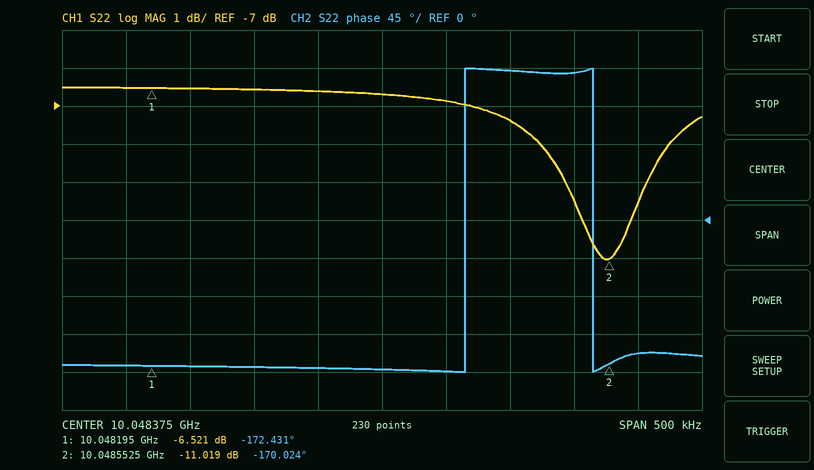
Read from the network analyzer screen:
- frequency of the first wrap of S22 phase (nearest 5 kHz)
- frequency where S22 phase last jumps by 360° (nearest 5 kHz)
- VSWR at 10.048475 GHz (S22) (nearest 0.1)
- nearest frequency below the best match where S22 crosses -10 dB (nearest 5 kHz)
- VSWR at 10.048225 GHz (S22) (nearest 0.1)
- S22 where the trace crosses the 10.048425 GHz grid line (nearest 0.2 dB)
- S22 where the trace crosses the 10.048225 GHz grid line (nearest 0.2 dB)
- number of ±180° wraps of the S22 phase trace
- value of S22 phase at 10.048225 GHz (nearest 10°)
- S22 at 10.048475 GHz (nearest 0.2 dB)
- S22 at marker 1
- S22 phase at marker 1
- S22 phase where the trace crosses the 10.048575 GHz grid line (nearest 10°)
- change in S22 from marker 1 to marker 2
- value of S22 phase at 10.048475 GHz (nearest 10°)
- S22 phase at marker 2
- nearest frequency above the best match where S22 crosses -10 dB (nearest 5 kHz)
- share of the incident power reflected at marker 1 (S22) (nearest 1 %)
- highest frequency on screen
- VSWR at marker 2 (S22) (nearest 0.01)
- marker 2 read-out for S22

10.048440 GHz
10.048540 GHz
2.5
10.048530 GHz
2.8
-6.8 dB
-6.6 dB
2
-170°
-7.4 dB
-6.521 dB
-172.431°
-160°
-4.498 dB
180°
-170.024°
10.048570 GHz
22 %
10.048625 GHz
1.78
-11.019 dB
